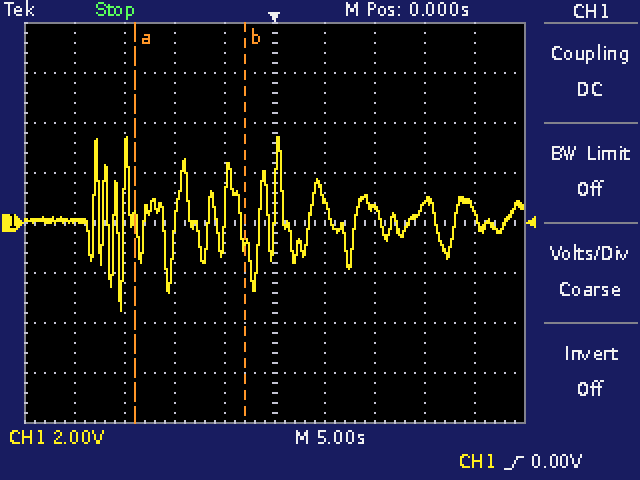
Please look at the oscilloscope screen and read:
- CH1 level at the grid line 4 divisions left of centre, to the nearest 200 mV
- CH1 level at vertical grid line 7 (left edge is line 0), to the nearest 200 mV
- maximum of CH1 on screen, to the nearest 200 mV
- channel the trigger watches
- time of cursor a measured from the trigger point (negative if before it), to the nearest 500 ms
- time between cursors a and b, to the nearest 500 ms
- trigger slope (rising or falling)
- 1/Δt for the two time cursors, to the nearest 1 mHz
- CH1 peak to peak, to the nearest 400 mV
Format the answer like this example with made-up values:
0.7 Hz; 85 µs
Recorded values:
0.0 V; 600 mV; 3.4 V; CH1; -14.0 s; 11.0 s; rising; 91 mHz; 6.8 V
